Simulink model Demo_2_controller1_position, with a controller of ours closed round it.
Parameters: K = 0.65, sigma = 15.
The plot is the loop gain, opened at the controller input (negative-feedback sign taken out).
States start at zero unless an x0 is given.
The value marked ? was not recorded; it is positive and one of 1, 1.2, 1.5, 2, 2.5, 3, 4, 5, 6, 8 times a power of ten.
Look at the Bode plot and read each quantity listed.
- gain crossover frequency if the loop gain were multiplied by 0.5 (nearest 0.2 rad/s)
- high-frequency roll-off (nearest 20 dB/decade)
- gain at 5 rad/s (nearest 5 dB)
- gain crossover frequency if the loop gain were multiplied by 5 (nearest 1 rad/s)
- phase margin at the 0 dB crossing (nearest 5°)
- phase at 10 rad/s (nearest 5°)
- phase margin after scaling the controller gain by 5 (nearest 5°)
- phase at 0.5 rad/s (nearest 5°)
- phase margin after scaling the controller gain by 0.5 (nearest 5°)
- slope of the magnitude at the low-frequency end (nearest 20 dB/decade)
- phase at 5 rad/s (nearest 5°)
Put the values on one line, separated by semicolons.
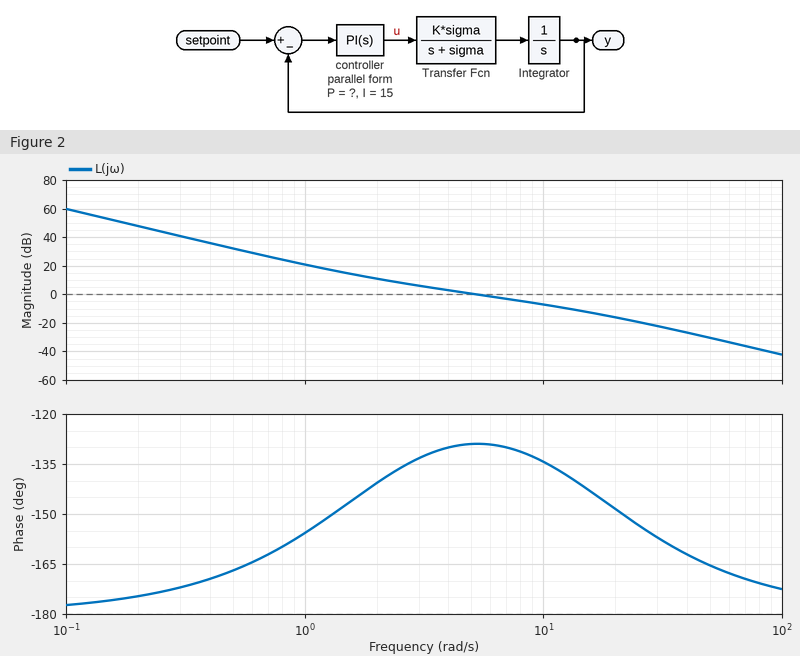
3.0 rad/s; -40 dB/decade; 0 dB; 17 rad/s; 50°; -135°; 35°; -165°; 45°; -40 dB/decade; -130°
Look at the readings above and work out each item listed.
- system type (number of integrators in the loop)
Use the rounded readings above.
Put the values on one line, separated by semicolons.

2
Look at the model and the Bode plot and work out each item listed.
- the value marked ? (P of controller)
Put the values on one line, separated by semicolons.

8
